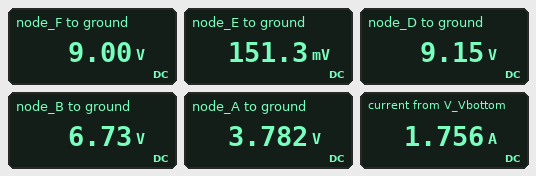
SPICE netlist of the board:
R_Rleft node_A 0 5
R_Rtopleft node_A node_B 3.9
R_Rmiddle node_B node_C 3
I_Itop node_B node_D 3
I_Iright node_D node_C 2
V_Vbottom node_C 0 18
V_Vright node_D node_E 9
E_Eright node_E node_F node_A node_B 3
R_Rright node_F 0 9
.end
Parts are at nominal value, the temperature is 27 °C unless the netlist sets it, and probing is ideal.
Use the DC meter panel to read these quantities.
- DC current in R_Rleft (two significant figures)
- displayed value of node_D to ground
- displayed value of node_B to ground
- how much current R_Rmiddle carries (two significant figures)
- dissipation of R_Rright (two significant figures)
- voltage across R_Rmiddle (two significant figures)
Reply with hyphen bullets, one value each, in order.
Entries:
- 760 mA
- 9.15 V
- 6.73 V
- 3.8 A
- 9.0 W
- 11 V
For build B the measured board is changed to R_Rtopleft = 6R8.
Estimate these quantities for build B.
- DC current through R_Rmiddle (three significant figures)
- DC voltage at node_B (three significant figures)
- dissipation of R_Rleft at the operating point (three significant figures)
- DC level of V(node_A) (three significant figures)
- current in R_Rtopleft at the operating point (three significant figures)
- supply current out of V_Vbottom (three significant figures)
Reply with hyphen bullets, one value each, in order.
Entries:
- 3.61 A
- 7.18 V
- 1.85 W
- 3.04 V
- 608 mA
- 1.61 A
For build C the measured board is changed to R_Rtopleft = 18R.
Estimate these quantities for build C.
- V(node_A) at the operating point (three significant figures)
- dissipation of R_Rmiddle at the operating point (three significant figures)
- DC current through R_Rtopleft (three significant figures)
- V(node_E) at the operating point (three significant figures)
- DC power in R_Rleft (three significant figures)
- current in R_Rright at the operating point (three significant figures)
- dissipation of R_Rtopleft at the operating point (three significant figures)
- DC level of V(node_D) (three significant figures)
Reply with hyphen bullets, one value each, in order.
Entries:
- 1.73 V
- 33.6 W
- 346 mA
- -9.69 V
- 599 mW
- 1.00 A
- 2.16 W
- -692 mV
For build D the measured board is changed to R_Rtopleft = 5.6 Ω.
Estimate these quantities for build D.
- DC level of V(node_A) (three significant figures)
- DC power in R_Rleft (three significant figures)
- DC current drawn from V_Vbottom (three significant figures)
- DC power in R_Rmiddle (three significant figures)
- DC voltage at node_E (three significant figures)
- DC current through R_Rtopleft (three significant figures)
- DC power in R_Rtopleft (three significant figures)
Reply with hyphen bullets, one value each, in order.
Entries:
- 3.31 V
- 2.19 W
- 1.66 A
- 40.2 W
- -2.12 V
- 662 mA
- 2.45 W
